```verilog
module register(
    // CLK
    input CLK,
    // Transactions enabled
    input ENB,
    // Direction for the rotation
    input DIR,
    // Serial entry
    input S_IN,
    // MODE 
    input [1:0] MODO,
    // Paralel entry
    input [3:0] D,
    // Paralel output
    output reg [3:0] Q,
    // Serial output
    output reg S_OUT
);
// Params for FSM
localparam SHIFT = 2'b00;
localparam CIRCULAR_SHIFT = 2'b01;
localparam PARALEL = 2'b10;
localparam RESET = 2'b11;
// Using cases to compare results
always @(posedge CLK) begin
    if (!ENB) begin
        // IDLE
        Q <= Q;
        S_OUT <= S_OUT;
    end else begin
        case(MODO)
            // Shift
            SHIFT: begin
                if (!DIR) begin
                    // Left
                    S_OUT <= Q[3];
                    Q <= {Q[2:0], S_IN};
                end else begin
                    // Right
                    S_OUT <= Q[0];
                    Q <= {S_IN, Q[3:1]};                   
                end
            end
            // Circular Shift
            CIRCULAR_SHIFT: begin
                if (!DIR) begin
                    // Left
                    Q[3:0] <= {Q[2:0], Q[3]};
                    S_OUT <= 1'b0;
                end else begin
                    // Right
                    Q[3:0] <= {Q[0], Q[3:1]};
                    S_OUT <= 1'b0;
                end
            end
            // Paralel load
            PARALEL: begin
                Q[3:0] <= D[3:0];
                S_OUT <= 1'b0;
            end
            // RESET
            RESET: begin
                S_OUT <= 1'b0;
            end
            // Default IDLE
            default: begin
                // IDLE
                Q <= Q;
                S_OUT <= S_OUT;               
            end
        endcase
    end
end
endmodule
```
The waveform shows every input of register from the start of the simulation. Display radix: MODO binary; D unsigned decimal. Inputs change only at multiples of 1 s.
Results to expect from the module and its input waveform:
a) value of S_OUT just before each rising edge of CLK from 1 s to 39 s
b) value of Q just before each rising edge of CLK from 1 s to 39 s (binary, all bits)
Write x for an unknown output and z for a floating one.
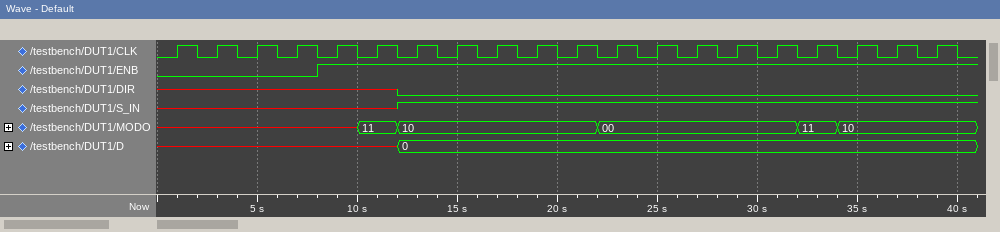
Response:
x x x x x x 0 0 0 0 0 0 0 0 0 0 1 0 0 0
x, x, x, x, x, x, x, 0000, 0000, 0000, 0000, 0000, 0001, 0011, 0111, 1111, 1111, 1111, 0000, 0000
